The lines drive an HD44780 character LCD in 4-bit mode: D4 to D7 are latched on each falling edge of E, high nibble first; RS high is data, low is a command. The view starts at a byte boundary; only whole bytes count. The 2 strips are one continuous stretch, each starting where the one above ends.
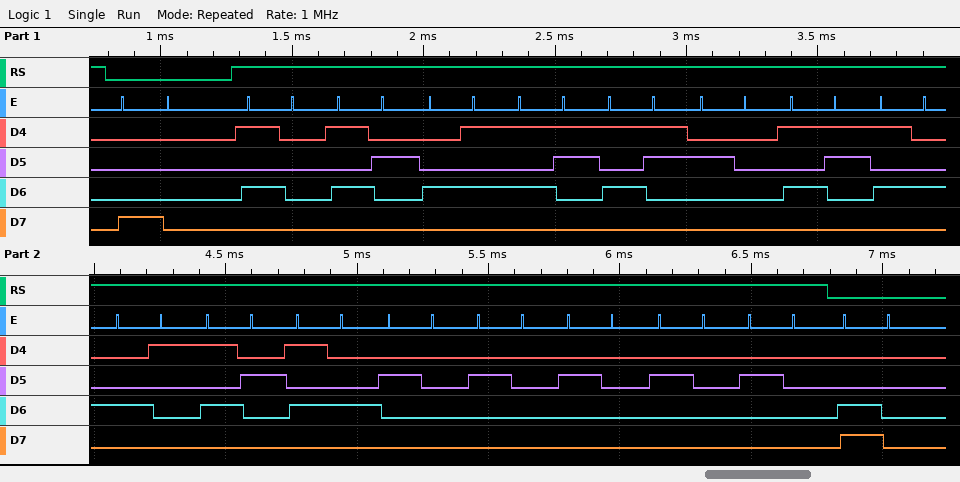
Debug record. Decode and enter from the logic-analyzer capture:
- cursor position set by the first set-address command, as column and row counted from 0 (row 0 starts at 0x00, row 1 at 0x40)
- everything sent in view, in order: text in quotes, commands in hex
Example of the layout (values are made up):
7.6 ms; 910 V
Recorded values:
column 0, row 0; 0x80 "PRESS START     " 0xC0
